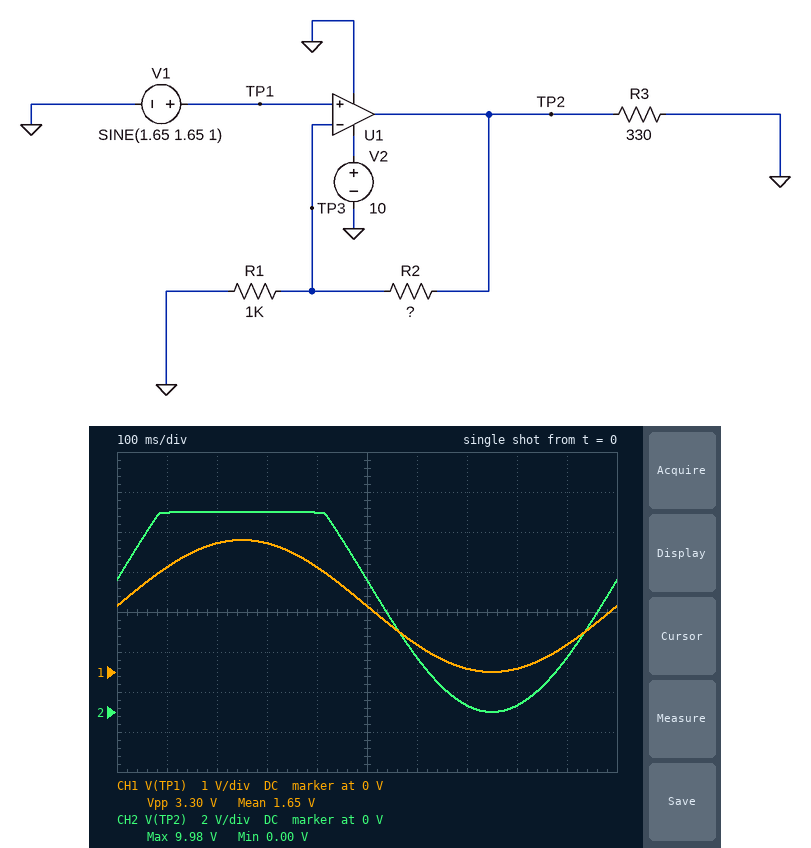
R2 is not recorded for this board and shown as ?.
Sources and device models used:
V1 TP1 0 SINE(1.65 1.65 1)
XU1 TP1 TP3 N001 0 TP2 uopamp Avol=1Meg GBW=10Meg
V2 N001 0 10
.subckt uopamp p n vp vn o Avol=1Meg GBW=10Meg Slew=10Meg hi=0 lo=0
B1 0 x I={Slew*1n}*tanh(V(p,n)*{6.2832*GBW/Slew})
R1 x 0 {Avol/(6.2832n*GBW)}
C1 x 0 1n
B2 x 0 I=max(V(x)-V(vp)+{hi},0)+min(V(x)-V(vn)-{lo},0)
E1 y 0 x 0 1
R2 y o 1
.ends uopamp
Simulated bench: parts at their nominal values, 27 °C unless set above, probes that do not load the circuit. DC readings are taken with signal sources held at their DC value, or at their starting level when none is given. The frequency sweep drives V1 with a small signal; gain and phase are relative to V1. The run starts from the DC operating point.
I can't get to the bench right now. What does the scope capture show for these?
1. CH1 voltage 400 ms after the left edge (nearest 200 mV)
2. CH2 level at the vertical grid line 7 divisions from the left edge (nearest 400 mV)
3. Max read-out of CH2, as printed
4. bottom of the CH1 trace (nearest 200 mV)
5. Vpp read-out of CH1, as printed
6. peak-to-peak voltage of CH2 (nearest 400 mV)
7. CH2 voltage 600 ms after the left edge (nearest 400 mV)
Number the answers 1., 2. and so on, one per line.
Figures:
1. 2.6 V
2. 400 mV
3. 9.98 V
4. 0 V
5. 3.30 V
6. 10.0 V
7. 2.8 V
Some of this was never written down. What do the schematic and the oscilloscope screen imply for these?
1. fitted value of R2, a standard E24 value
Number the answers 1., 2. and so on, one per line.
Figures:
1. 3 kΩ
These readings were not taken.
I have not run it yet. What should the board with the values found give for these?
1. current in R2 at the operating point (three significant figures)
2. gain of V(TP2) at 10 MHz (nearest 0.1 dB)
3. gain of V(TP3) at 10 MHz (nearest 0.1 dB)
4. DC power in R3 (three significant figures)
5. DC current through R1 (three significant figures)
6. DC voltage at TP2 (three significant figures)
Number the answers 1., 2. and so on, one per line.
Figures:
1. 1.65 mA
2. -0.3 dB
3. -12.3 dB
4. 132 mW
5. 1.65 mA
6. 6.60 V
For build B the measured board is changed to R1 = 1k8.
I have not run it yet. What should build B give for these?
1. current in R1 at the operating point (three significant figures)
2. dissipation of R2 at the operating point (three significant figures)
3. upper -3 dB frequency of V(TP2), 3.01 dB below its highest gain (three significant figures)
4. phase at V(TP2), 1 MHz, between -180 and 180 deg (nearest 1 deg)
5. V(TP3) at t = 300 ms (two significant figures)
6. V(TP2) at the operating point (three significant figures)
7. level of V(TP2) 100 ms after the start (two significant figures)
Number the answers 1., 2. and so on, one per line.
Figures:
1. 917 µA
2. 2.52 mW
3. 3.74 MHz
4. -15 deg
5. 3.2 V
6. 4.40 V
7. 7.0 V
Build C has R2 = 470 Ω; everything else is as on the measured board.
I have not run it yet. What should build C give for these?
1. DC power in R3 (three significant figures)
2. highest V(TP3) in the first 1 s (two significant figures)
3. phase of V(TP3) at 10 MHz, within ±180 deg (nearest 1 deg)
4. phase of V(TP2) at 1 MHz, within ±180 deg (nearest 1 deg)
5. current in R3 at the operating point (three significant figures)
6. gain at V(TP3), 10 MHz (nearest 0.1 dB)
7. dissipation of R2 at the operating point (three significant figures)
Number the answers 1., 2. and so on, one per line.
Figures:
1. 17.8 mW
2. 3.3 V
3. -56 deg
4. -8 deg
5. 7.35 mA
6. -5.0 dB
7. 1.28 mW
